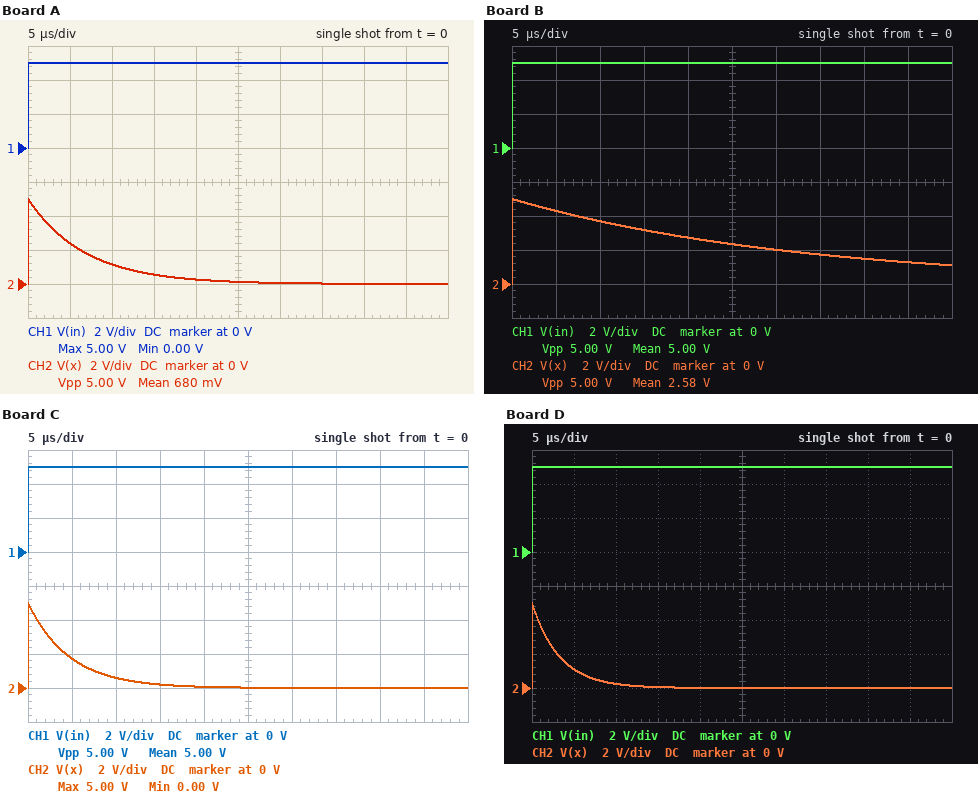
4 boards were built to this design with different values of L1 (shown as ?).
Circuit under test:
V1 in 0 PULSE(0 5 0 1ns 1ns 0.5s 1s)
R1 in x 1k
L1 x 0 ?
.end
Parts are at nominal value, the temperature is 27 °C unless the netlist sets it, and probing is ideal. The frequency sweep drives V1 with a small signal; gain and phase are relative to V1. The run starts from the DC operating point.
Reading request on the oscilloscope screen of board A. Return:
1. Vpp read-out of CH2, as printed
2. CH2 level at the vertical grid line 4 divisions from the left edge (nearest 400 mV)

5.00 V
400 mV
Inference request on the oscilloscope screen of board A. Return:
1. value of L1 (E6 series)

6.8 mH
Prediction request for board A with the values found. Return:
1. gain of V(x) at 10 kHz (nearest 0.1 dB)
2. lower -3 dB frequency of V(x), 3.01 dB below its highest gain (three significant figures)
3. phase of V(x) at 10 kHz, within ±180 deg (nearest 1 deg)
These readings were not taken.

-8.1 dB
23.4 kHz
67 deg
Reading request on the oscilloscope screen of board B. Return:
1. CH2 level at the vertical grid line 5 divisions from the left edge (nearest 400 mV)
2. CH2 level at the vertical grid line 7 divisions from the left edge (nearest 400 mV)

2.4 V
1.6 V
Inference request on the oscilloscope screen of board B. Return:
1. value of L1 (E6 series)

33 mH
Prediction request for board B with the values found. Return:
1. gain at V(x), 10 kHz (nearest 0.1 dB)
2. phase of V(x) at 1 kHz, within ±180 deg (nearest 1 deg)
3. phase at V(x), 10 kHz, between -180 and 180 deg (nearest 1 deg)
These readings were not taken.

-0.9 dB
78 deg
26 deg
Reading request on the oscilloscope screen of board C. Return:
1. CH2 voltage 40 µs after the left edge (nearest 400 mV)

0 V
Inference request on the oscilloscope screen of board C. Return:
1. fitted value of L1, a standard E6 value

4.7 mH
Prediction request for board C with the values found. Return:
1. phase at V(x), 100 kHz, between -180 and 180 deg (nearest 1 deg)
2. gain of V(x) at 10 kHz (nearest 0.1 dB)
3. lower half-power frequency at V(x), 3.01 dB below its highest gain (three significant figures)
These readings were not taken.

19 deg
-11.0 dB
33.9 kHz
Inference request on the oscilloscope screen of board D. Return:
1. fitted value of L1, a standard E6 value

3.3 mH
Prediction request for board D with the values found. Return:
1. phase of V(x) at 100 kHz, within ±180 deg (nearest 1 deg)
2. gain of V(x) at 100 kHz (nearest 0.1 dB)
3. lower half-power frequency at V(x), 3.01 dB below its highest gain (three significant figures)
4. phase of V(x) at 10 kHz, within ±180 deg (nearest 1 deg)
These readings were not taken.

26 deg
-0.9 dB
48.2 kHz
78 deg
